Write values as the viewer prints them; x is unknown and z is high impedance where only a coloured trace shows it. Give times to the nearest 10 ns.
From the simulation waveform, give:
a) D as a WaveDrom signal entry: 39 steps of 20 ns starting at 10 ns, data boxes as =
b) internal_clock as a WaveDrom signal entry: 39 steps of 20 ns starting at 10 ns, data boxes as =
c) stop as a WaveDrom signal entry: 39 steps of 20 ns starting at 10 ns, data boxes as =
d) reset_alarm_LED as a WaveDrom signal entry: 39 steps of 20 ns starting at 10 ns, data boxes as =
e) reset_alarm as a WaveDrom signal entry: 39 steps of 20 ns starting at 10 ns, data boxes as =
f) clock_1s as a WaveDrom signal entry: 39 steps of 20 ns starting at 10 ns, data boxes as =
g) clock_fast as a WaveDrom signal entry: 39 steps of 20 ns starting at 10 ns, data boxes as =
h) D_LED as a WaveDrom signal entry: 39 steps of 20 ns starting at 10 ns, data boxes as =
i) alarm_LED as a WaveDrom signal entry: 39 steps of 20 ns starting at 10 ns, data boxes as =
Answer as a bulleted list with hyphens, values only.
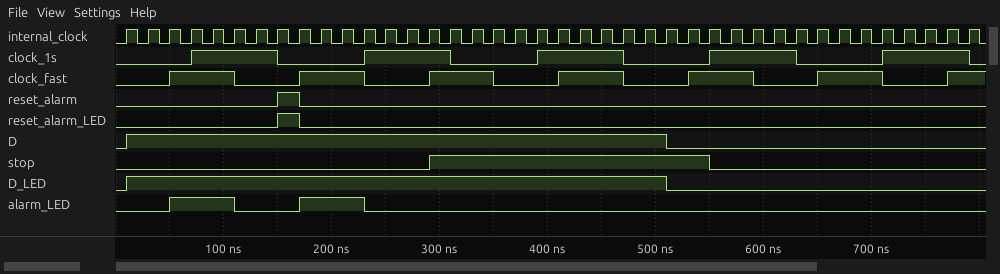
- {name: 'D', wave: '1........................0.............'}
- {name: 'internal_clock', wave: 'p......................................'}
- {name: 'stop', wave: '0.............1............0...........'}
- {name: 'reset_alarm_LED', wave: '0......10..............................'}
- {name: 'reset_alarm', wave: '0......10..............................'}
- {name: 'clock_1s', wave: '0..1...0...1...0...1...0...1...0...1...'}
- {name: 'clock_fast', wave: '0.1..0..1..0..1..0..1..0..1..0..1..0..1'}
- {name: 'D_LED', wave: '1........................0.............'}
- {name: 'alarm_LED', wave: '0.1..0..1..0...........................'}
